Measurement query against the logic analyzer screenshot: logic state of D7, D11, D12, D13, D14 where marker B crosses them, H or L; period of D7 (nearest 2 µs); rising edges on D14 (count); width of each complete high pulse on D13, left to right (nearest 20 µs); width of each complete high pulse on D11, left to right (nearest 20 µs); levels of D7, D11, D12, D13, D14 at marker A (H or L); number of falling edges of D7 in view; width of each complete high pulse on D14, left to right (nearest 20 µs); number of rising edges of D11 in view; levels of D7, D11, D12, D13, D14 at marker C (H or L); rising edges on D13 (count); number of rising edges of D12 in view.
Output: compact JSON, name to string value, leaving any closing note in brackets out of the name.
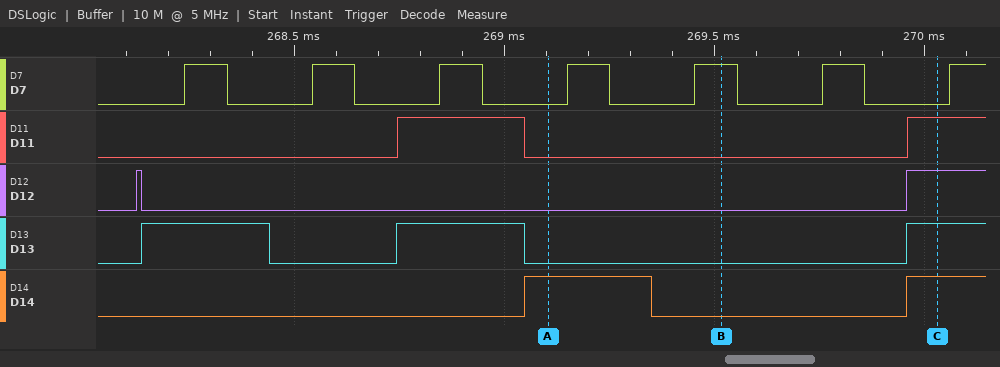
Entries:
{"logic state of D7, D11, D12, D13, D14 where marker B crosses them, H or L": "D7=H, D11=L, D12=L, D13=L, D14=L", "period of D7": "304 µs", "rising edges on D14": "2", "width of each complete high pulse on D13, left to right": "300 µs, 300 µs", "width of each complete high pulse on D11, left to right": "300 µs", "levels of D7, D11, D12, D13, D14 at marker A": "D7=L, D11=L, D12=L, D13=L, D14=H", "number of falling edges of D7 in view": "6", "width of each complete high pulse on D14, left to right": "300 µs", "number of rising edges of D11 in view": "2", "levels of D7, D11, D12, D13, D14 at marker C": "D7=L, D11=H, D12=H, D13=H, D14=H", "rising edges on D13": "3", "number of rising edges of D12 in view": "2"}
